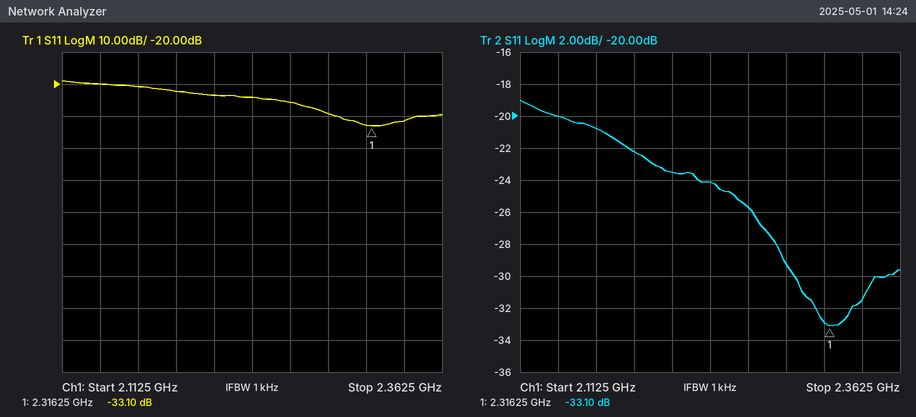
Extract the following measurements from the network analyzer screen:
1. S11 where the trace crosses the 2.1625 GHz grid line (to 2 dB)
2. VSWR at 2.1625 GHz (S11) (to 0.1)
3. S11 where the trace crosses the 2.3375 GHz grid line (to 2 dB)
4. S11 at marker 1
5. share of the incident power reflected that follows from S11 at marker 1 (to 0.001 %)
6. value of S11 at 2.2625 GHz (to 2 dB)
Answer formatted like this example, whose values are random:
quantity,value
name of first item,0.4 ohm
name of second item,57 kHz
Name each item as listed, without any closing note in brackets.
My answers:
quantity,value
S11 where the trace crosses the 2.1625 GHz grid line,-20 dB
VSWR at 2.1625 GHz (S11),1.2
S11 where the trace crosses the 2.3375 GHz grid line,-32 dB
S11 at marker 1,-33.10 dB
share of the incident power reflected that follows from S11 at marker 1,0.049 %
value of S11 at 2.2625 GHz,-26 dB
